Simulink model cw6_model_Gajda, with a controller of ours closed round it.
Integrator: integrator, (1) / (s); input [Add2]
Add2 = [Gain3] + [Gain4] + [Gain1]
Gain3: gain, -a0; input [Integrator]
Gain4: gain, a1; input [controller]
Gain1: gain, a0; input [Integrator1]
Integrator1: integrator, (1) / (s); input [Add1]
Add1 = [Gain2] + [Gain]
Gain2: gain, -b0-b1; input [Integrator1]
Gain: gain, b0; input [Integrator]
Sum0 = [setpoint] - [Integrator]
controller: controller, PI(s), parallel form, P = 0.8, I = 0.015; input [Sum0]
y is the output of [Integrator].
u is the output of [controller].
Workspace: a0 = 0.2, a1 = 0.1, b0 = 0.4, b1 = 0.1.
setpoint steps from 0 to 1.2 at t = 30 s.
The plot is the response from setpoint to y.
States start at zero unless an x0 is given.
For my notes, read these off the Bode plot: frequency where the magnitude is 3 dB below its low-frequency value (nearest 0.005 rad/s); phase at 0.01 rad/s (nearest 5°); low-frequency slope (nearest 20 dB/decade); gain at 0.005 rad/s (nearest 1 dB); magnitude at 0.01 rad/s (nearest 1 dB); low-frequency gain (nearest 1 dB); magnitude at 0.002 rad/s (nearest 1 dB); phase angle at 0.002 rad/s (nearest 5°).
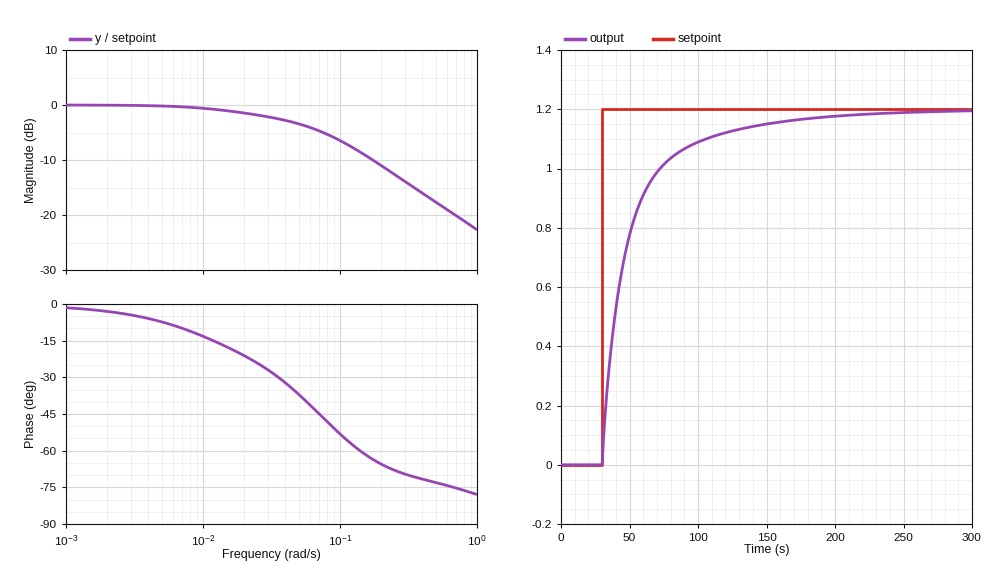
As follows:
0.045 rad/s
-15°
0 dB/decade
0 dB
-1 dB
0 dB
0 dB
-5°
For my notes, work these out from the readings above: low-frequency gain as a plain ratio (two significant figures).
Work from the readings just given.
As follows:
1.0
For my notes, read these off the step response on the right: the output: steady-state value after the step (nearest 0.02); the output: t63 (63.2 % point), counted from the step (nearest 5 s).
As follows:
1.20
20 s
